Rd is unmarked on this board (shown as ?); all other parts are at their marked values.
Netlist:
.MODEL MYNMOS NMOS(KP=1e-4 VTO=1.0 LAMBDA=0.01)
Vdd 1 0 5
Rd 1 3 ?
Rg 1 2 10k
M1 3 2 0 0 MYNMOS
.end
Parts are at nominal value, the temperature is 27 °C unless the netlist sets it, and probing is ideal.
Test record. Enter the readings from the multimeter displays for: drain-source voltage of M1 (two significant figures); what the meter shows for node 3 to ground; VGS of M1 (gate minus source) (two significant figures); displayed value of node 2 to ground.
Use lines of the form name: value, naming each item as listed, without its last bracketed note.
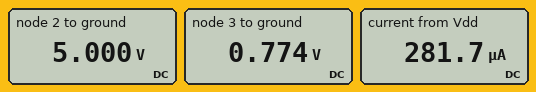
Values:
drain-source voltage of M1: 770 mV
what the meter shows for node 3 to ground: 0.774 V
VGS of M1 (gate minus source): 5.0 V
displayed value of node 2 to ground: 5.000 V
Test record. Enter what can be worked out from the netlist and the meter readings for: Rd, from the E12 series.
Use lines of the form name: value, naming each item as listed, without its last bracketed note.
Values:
Rd, from the E12 series: 15 kΩ
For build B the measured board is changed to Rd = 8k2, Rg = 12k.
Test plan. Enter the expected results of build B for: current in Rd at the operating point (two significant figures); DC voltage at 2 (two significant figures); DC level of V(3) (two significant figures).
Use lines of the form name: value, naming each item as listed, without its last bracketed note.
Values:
current in Rd at the operating point: 450 µA
DC voltage at 2: 5.0 V
DC level of V(3): 1.3 V
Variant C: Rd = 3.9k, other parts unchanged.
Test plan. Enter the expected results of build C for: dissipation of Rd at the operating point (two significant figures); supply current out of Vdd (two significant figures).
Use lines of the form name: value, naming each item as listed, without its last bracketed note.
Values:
dissipation of Rd at the operating point: 1.8 mW
supply current out of Vdd: 680 µA
